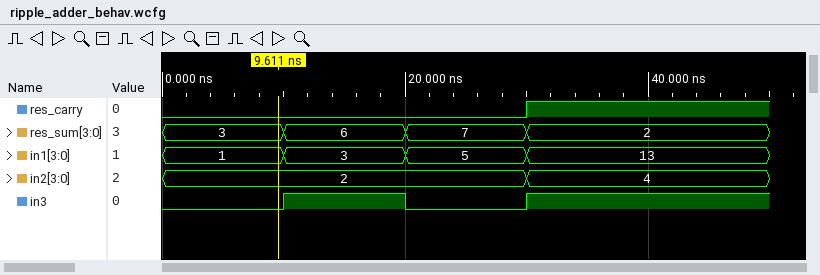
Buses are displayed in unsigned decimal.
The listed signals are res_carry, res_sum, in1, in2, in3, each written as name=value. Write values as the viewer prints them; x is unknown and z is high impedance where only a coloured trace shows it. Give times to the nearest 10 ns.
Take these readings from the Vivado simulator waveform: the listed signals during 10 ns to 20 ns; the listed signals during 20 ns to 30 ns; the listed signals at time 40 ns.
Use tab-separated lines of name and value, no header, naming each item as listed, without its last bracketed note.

the listed signals during 10 ns to 20 ns	res_carry=0, res_sum=6, in1=3, in2=2, in3=1
the listed signals during 20 ns to 30 ns	res_carry=0, res_sum=7, in1=5, in2=2, in3=0
the listed signals at time 40 ns	res_carry=1, res_sum=2, in1=13, in2=4, in3=1
